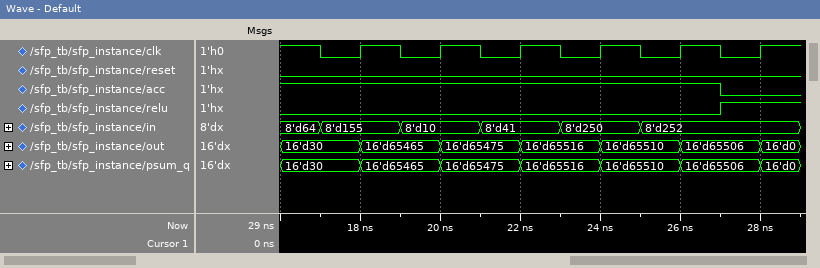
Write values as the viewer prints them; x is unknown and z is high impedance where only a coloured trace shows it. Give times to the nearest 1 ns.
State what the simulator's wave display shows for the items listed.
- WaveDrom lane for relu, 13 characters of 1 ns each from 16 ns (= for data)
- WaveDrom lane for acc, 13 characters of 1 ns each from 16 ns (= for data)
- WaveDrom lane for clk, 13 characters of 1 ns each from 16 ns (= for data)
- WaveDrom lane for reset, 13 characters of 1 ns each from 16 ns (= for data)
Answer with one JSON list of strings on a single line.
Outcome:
["{name: 'relu', wave: '0..........1.'}", "{name: 'acc', wave: '1..........0.'}", "{name: 'clk', wave: '1010101010101'}", "{name: 'reset', wave: '0............'}"]
